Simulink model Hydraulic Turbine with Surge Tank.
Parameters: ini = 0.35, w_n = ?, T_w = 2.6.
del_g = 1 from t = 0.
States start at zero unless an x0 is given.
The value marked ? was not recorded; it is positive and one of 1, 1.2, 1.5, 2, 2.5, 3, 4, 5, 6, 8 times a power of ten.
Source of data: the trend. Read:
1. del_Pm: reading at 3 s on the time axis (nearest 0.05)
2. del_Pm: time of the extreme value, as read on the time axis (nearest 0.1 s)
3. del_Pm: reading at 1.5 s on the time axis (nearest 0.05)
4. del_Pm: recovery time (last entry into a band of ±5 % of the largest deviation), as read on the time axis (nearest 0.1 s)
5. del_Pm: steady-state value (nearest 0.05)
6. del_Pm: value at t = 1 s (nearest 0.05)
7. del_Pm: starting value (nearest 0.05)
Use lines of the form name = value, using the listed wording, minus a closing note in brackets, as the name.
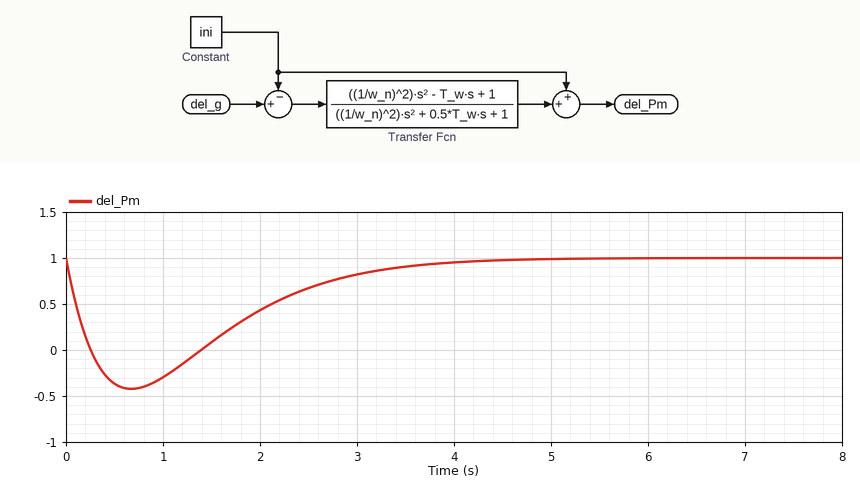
del_Pm: reading at 3 s on the time axis = 0.80
del_Pm: time of the extreme value, as read on the time axis = 0.7 s
del_Pm: reading at 1.5 s on the time axis = 0.10
del_Pm: recovery time (last entry into a band of ±5 % of the largest deviation), as read on the time axis = 3.7 s
del_Pm: steady-state value = 1.00
del_Pm: value at t = 1 s = -0.30
del_Pm: starting value = 1.00
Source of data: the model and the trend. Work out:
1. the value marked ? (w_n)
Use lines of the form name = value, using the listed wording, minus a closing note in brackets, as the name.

the value marked ? = 1.5
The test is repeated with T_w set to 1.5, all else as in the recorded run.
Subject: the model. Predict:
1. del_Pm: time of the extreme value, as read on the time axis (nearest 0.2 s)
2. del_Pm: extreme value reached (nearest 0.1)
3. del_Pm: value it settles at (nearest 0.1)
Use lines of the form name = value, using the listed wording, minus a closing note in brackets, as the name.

del_Pm: time of the extreme value, as read on the time axis = 0.8 s
del_Pm: extreme value reached = -0.1
del_Pm: value it settles at = 1.0
